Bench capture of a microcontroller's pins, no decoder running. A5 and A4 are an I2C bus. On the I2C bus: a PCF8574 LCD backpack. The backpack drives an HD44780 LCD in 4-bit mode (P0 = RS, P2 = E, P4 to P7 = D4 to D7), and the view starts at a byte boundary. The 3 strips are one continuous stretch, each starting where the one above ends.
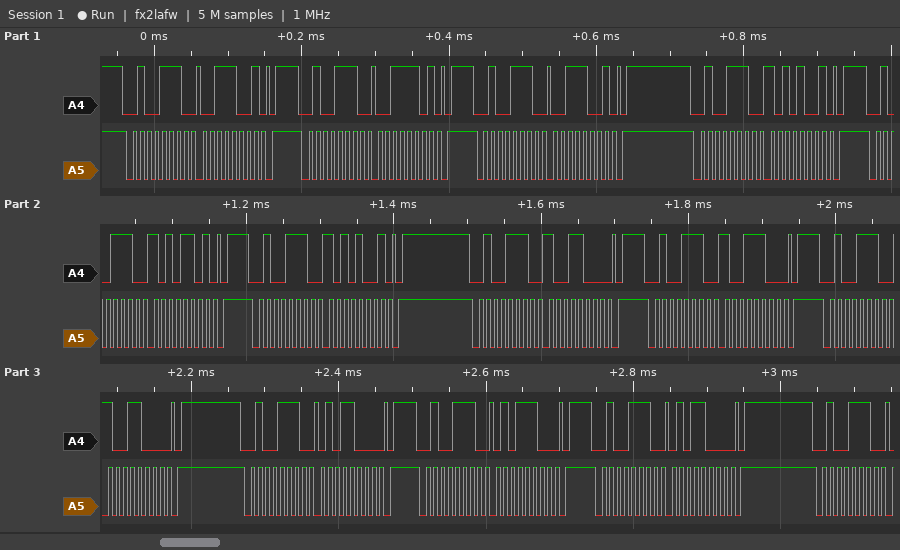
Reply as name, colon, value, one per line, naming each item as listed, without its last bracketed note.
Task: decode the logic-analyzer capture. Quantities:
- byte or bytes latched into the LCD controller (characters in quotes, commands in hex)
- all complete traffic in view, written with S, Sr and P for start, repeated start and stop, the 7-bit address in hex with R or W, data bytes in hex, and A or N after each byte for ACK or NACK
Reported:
byte or bytes latched into the LCD controller: ':' 0x95
all complete traffic in view, written with S, Sr and P for start, repeated start and stop, the 7-bit address in hex with R or W, data bytes in hex, and A or N after each byte for ACK or NACK: S 27W A 39 A P S 27W A 3D A P S 27W A 39 A P S 27W A A9 A P S 27W A AD A P S 27W A A9 A P S 27W A 98 A P S 27W A 9C A P S 27W A 98 A P S 27W A 58 A P S 27W A 5C A P S 27W A 58 A P S 27W A
